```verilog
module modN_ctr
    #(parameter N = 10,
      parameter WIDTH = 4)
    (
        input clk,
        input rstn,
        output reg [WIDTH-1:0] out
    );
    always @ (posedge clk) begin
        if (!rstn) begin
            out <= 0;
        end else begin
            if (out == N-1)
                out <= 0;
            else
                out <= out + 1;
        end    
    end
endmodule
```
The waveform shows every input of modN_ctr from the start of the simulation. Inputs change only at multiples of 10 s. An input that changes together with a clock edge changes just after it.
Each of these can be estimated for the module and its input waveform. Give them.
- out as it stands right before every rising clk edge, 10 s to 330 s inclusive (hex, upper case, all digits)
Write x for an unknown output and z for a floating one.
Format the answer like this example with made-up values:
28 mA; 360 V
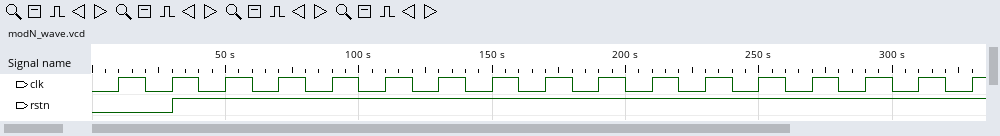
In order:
x, 0, 0, 1, 2, 3, 4, 5, 6, 7, 8, 9, 0, 1, 2, 3, 4
